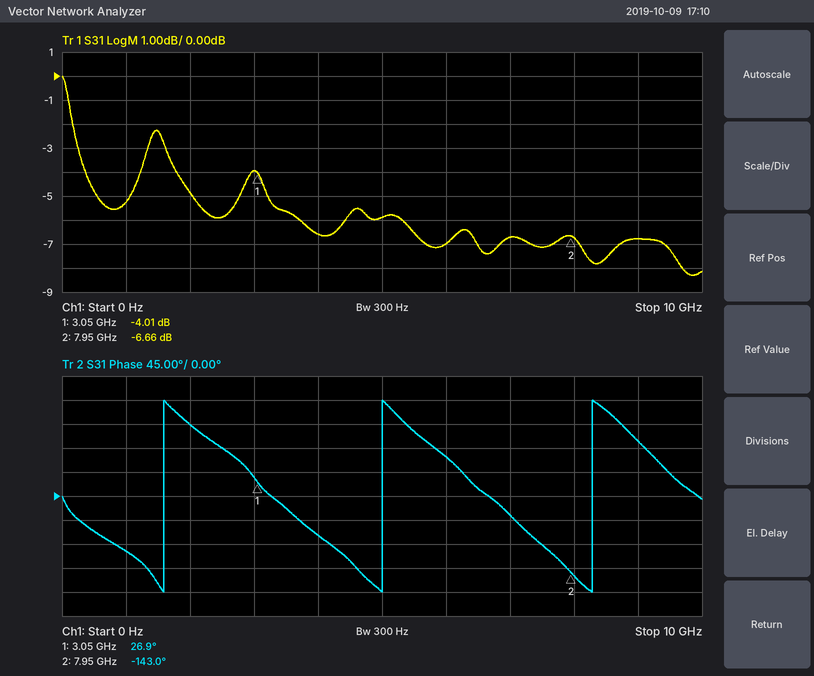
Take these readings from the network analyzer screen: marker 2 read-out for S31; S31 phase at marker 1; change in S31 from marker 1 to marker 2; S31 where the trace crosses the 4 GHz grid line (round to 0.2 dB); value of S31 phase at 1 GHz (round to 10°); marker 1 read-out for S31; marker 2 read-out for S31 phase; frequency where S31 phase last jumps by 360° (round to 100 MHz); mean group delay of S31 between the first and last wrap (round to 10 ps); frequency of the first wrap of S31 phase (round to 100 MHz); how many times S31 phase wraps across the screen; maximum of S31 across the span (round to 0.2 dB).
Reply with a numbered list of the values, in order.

1. -6.66 dB
2. 26.9°
3. -2.65 dB
4. -6.6 dB
5. -100°
6. -4.01 dB
7. -143.0°
8. 8.3 GHz
9. 300 ps
10. 1.6 GHz
11. 3
12. 0.0 dB
